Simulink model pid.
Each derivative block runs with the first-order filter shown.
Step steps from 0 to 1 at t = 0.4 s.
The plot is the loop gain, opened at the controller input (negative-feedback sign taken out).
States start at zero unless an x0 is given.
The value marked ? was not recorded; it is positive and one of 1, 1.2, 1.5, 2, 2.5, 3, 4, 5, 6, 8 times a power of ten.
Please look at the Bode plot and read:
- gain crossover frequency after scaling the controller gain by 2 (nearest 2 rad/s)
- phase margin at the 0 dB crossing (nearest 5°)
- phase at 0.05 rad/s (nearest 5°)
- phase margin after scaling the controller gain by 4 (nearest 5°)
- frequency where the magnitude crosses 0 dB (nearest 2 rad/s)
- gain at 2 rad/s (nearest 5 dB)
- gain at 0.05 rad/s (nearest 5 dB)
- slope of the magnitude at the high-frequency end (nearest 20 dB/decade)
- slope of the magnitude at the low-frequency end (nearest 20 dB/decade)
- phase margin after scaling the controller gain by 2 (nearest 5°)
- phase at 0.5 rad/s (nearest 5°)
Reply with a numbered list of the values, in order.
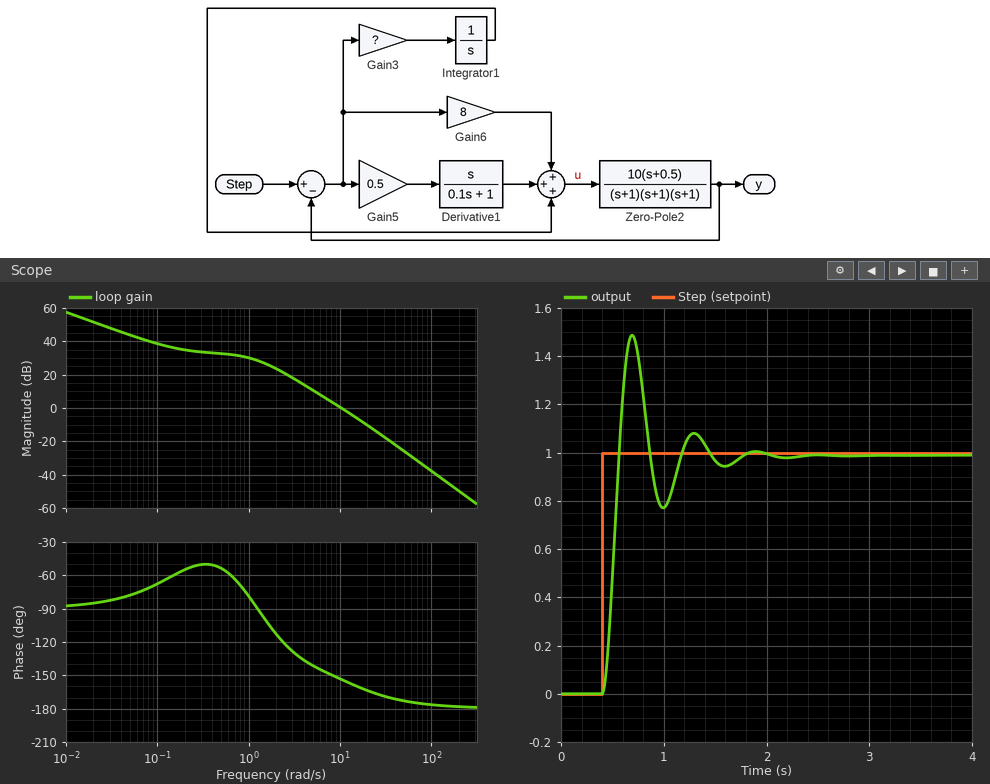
1. 16 rad/s
2. 25°
3. -80°
4. 15°
5. 10 rad/s
6. 25 dB
7. 45 dB
8. -40 dB/decade
9. -20 dB/decade
10. 20°
11. -55°
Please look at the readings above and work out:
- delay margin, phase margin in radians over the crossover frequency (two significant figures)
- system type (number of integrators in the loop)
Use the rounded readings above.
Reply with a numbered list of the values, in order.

1. 0.044 s
2. 1
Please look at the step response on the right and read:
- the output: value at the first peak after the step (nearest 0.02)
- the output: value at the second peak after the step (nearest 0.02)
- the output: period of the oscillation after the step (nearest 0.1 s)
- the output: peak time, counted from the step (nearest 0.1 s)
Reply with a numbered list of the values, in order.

1. 1.48
2. 1.08
3. 0.6 s
4. 0.3 s
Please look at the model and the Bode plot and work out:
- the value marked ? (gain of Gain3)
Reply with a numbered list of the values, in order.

1. 1.5
